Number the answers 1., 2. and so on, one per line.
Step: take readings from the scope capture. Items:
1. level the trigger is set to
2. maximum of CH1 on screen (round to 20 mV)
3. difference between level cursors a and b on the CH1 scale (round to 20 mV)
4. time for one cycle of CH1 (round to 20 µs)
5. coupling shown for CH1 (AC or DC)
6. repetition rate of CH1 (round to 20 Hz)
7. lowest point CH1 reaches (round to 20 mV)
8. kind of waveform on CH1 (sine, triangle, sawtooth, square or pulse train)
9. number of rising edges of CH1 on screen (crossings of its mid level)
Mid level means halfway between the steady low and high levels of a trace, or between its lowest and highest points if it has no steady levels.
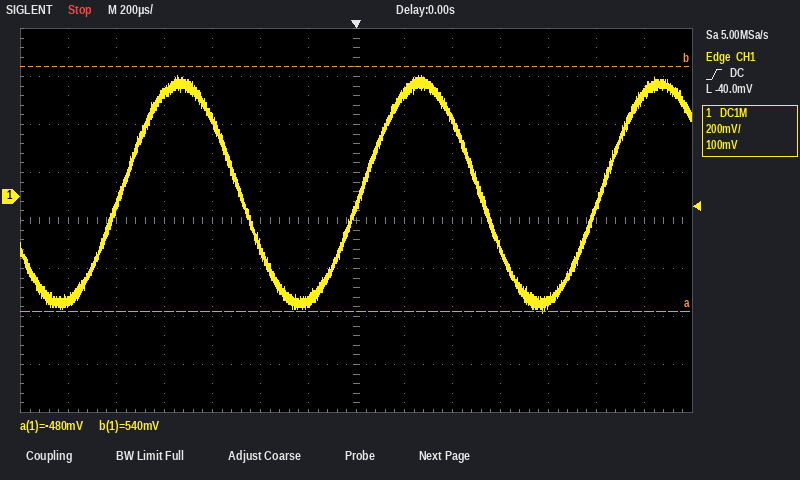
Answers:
1. -40.0 mV
2. 500 mV
3. 1.02 V
4. 1.00 ms
5. DC
6. 1.00 kHz
7. -480 mV
8. sine
9. 3
